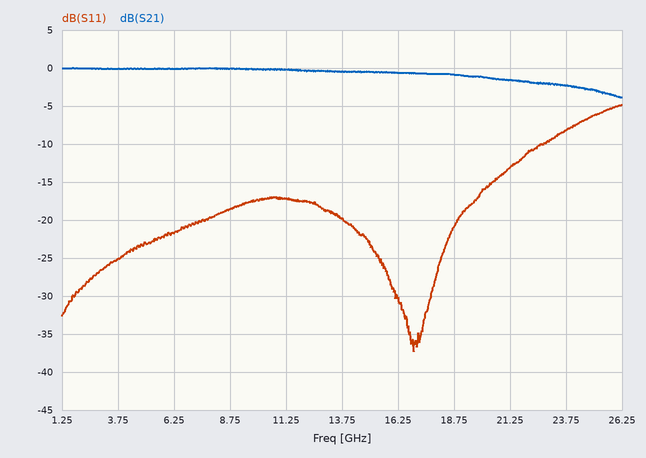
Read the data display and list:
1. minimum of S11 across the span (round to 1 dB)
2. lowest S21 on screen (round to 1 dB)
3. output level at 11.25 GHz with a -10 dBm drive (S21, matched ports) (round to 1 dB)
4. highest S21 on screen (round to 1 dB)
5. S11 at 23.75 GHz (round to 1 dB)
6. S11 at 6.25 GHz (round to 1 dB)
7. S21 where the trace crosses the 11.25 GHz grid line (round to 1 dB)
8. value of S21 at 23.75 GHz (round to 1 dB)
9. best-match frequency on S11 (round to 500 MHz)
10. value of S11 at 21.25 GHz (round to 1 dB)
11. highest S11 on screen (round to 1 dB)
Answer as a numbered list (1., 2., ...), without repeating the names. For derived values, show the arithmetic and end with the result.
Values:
1. -37 dB
2. -4 dB
3. -10 dBm + (0 dB) = -10 dBm
4. 0 dB
5. -8 dB
6. -22 dB
7. 0 dB
8. -2 dB
9. 17.0 GHz
10. -13 dB
11. -5 dB
